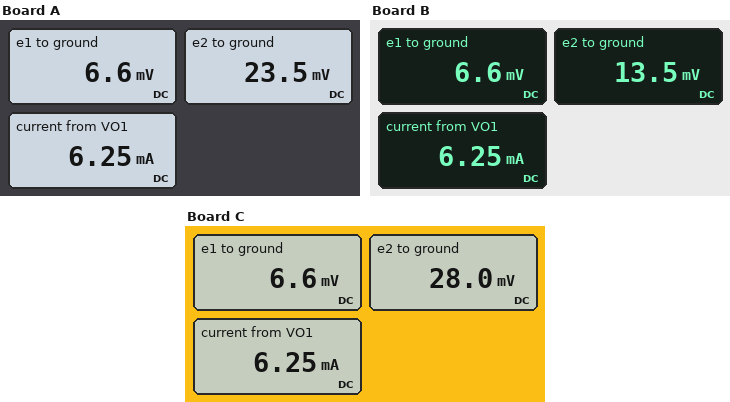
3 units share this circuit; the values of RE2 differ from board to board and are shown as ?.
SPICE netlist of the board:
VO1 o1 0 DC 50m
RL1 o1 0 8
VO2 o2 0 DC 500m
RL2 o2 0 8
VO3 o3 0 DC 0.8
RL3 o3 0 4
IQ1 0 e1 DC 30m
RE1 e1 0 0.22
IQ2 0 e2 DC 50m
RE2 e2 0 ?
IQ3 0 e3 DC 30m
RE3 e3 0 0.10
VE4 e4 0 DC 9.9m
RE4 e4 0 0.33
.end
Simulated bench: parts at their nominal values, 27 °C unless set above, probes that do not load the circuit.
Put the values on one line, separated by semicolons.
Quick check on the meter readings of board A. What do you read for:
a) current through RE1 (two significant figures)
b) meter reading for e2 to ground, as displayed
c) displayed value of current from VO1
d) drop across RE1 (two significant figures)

30 mA; 23.5 mV; 6.25 mA; 6.6 mV
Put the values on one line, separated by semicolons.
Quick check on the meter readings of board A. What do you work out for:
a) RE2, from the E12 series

0.47 Ω
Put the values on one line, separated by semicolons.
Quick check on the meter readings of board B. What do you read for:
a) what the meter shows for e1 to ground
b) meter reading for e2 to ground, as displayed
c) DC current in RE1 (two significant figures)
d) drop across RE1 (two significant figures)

6.6 mV; 13.5 mV; 30 mA; 6.6 mV
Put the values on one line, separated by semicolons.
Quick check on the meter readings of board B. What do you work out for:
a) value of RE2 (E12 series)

0.27 Ω
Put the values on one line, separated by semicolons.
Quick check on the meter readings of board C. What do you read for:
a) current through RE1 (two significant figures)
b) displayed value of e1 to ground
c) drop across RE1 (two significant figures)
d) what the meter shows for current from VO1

30 mA; 6.6 mV; 6.6 mV; 6.25 mA
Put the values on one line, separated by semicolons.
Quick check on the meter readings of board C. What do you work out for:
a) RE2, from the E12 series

0.56 Ω
